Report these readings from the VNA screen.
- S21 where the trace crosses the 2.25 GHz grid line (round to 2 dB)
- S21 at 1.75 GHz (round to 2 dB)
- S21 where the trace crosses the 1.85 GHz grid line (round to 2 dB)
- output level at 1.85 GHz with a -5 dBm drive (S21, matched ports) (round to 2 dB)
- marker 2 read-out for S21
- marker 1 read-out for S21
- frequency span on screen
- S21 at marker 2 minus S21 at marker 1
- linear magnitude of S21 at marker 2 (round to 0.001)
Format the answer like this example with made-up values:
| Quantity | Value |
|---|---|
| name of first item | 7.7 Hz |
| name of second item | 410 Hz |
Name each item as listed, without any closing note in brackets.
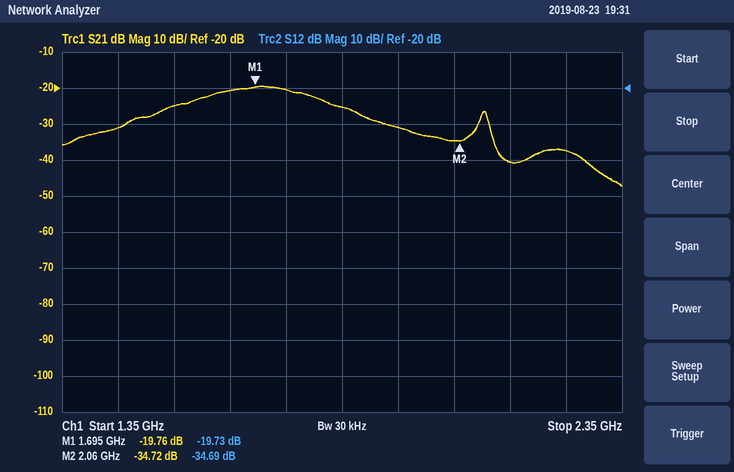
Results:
| Quantity | Value |
|---|---|
| S21 where the trace crosses the 2.25 GHz grid line | -38 dB |
| S21 at 1.75 GHz | -20 dB |
| S21 where the trace crosses the 1.85 GHz grid line | -26 dB |
| output level at 1.85 GHz with a -5 dBm drive (S21, matched ports) | -30 dBm |
| marker 2 read-out for S21 | -34.72 dB |
| marker 1 read-out for S21 | -19.76 dB |
| frequency span on screen | 1 GHz |
| S21 at marker 2 minus S21 at marker 1 | -14.96 dB |
| linear magnitude of S21 at marker 2 | 0.018 |
